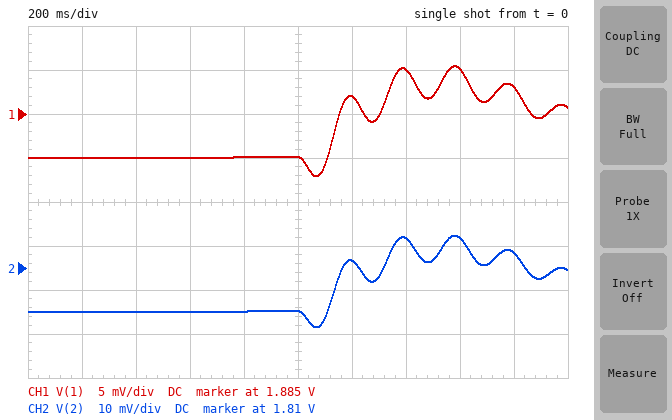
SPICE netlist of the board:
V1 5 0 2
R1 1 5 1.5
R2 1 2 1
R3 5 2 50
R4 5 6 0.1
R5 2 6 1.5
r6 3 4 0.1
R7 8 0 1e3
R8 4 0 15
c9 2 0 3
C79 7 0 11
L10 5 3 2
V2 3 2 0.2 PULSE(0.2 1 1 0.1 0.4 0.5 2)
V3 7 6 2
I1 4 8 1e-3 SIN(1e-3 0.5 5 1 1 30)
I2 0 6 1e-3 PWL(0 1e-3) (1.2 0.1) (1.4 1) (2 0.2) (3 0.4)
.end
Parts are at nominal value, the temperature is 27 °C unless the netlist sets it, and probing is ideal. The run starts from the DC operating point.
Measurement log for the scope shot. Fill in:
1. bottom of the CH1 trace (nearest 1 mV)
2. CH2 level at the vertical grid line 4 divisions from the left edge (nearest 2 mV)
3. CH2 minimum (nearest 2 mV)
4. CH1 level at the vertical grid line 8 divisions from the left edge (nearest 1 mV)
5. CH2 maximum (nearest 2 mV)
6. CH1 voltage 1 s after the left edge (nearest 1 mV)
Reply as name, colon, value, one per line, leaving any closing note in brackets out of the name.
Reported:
bottom of the CH1 trace: 1.878 V
CH2 level at the vertical grid line 4 divisions from the left edge: 1.800 V
CH2 minimum: 1.796 V
CH1 level at the vertical grid line 8 divisions from the left edge: 1.890 V
CH2 maximum: 1.818 V
CH1 voltage 1 s after the left edge: 1.880 V
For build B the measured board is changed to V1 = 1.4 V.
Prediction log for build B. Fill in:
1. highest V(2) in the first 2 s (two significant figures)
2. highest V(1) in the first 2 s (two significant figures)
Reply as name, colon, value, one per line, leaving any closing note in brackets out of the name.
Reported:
highest V(2) in the first 2 s: 1.2 V
highest V(1) in the first 2 s: 1.3 V
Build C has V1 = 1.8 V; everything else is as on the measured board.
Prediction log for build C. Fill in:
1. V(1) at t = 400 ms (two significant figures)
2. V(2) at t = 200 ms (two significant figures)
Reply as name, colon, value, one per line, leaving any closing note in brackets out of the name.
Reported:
V(1) at t = 400 ms: 1.7 V
V(2) at t = 200 ms: 1.6 V
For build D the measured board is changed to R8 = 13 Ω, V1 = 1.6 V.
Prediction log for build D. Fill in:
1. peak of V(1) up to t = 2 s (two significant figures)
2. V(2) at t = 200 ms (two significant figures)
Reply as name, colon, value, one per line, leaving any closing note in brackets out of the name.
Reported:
peak of V(1) up to t = 2 s: 1.5 V
V(2) at t = 200 ms: 1.4 V
